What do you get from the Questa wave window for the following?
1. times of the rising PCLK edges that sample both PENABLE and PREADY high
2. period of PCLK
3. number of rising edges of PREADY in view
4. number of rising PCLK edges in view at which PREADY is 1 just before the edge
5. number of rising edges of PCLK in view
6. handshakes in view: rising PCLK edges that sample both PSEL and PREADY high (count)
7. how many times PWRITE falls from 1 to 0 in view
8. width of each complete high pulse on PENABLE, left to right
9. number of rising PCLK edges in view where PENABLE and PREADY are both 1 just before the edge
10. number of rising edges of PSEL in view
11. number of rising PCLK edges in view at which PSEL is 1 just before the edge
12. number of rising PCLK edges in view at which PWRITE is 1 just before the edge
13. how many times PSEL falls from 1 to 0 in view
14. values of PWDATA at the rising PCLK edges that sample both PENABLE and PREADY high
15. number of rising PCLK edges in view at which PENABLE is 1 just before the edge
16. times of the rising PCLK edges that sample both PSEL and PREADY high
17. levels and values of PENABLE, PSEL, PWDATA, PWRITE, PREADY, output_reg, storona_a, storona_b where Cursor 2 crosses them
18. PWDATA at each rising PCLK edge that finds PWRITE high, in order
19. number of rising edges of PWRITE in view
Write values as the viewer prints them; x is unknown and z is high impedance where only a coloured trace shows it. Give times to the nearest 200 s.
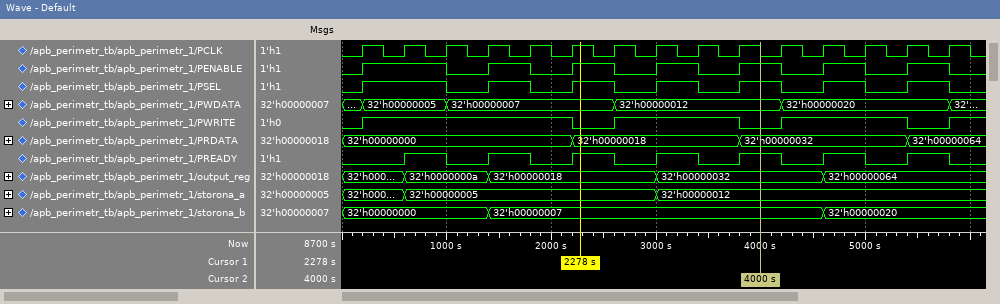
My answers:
1000 s, 1800 s, 2600 s, 3400 s, 4200 s, 5000 s, 5800 s
400 s
7
7
15
7
3
800 s, 400 s, 400 s, 400 s, 400 s, 400 s, 400 s
7
7
8
11
7
32'h00000005, 32'h00000007, 32'h00000007, 32'h00000012, 32'h00000012, 32'h00000020, 32'h00000020
8
1000 s, 1800 s, 2600 s, 3400 s, 4200 s, 5000 s, 5800 s
PENABLE=1, PSEL=1, PWDATA=32'h00000012, PWRITE=0, PREADY=1, output_reg=32'h00000032, storona_a=32'h00000012, storona_b=32'h00000007
32'h00000005, 32'h00000005, 32'h00000007, 32'h00000007, 32'h00000007, 32'h00000012, 32'h00000012, 32'h00000012, 32'h00000020, 32'h00000020, 32'h00000020
4
